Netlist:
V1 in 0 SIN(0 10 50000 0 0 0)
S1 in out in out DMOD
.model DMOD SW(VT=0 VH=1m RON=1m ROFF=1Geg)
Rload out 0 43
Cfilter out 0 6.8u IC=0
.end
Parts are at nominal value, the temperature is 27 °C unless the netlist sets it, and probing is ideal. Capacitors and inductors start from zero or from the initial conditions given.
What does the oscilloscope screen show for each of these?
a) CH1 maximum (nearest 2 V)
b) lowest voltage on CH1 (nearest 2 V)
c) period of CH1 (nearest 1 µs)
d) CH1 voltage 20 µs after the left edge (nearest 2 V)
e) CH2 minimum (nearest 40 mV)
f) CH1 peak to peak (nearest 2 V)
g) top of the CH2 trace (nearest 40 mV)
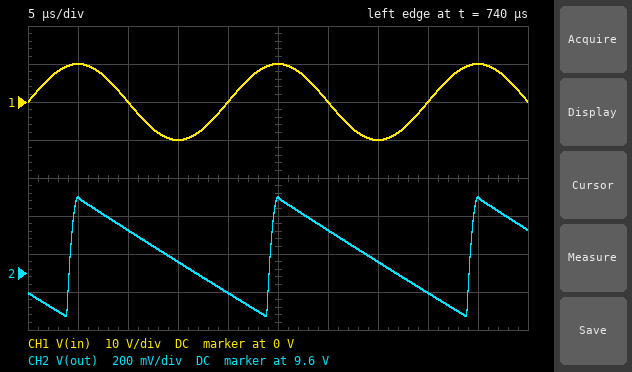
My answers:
10 V
-10 V
20 µs
0 V
9.36 V
20 V
10.00 V
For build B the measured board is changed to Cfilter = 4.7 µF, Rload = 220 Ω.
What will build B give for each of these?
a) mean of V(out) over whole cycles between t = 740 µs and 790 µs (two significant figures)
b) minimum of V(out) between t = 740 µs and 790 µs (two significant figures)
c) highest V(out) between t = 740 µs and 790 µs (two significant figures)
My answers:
9.9 V
9.8 V
10 V
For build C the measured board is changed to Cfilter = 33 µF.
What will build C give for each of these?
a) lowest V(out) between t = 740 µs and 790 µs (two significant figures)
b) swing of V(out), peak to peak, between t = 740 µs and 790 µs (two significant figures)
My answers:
9.9 V
140 mV
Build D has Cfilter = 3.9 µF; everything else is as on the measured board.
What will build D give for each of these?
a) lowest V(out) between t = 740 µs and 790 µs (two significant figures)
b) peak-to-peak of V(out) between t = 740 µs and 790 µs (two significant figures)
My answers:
8.9 V
1.1 V
